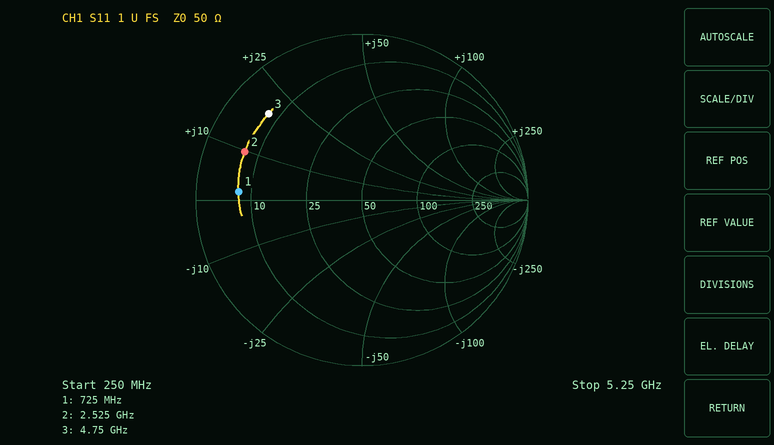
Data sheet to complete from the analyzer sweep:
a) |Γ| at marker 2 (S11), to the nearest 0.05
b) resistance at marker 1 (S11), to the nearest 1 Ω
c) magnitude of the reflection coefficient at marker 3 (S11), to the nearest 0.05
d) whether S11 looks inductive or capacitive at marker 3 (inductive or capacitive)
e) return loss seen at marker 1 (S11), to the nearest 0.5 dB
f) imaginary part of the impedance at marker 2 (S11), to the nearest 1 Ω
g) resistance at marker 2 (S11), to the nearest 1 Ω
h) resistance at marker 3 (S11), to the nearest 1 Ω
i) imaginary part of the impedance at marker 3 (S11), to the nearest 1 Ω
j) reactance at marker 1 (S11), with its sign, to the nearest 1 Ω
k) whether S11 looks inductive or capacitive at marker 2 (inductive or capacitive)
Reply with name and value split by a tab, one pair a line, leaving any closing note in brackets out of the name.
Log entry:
|Γ| at marker 2 (S11), to the nearest 0.05	0.75
resistance at marker 1 (S11), to the nearest 1 Ω	7 Ω
magnitude of the reflection coefficient at marker 3 (S11), to the nearest 0.05	0.75
whether S11 looks inductive or capacitive at marker 3	inductive
return loss seen at marker 1 (S11), to the nearest 0.5 dB	2.5 dB
imaginary part of the impedance at marker 2 (S11), to the nearest 1 Ω	+10 Ω
resistance at marker 2 (S11), to the nearest 1 Ω	7 Ω
resistance at marker 3 (S11), to the nearest 1 Ω	8 Ω
imaginary part of the impedance at marker 3 (S11), to the nearest 1 Ω	+19 Ω
reactance at marker 1 (S11), with its sign, to the nearest 1 Ω	+2 Ω
whether S11 looks inductive or capacitive at marker 2	inductive
